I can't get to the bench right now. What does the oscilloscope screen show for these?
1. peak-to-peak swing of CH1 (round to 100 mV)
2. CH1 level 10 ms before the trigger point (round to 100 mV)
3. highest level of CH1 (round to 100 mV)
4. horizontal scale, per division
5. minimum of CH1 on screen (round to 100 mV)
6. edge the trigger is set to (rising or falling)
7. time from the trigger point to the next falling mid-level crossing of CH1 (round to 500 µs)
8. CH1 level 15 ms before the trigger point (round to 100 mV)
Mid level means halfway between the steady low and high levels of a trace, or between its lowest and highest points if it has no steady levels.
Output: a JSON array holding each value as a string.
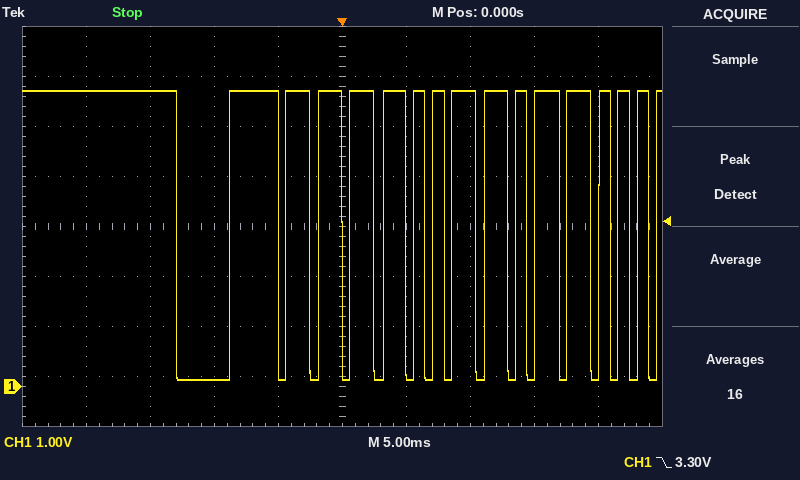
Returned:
["5.8 V", "100 mV", "5.9 V", "5 ms", "100 mV", "falling", "2.5 ms", "5.9 V"]
